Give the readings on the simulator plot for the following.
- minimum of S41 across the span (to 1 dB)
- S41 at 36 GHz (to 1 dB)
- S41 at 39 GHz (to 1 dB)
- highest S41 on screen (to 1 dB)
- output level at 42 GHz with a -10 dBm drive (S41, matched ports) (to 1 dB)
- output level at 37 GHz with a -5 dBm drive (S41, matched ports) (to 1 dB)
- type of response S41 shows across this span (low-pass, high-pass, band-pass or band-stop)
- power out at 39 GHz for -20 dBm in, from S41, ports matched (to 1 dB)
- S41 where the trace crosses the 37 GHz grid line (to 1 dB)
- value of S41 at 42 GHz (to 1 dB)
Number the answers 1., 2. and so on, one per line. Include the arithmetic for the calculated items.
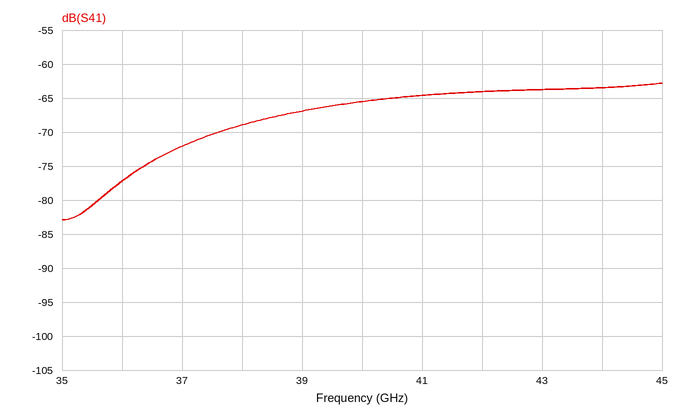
1. -83 dB
2. -77 dB
3. -67 dB
4. -63 dB
5. -10 dBm + (-64 dB) = -74 dBm
6. -5 dBm + (-72 dB) = -77 dBm
7. high-pass
8. -20 dBm + (-67 dB) = -87 dBm
9. -72 dB
10. -64 dB
